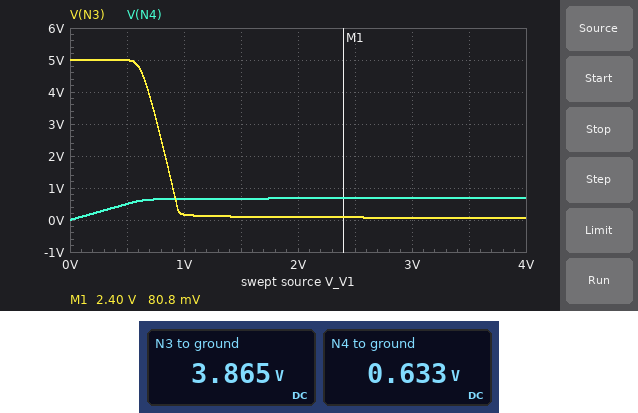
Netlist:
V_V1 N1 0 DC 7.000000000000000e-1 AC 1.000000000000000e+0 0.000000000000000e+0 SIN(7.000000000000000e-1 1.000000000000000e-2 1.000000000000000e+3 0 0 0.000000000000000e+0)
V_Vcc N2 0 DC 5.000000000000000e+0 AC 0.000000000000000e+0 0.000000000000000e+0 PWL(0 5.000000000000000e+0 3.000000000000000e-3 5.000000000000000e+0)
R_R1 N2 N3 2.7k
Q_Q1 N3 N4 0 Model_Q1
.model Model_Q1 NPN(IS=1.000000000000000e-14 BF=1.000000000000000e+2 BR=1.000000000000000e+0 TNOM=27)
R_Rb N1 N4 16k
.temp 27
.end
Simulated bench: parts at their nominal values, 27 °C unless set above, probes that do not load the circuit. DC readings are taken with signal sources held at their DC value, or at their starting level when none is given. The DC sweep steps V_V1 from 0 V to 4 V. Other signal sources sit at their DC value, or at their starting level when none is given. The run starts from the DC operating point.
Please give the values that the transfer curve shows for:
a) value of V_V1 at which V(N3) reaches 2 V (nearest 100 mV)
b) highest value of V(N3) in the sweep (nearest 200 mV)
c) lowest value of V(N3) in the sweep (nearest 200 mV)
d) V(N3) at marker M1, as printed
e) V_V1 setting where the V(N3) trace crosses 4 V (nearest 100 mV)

800 mV
5.0 V
0 V
80.8 mV
700 mV
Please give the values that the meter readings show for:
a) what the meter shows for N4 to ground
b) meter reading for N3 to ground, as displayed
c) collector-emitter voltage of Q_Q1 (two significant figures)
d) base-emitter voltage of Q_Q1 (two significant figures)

0.633 V
3.865 V
3.9 V
630 mV
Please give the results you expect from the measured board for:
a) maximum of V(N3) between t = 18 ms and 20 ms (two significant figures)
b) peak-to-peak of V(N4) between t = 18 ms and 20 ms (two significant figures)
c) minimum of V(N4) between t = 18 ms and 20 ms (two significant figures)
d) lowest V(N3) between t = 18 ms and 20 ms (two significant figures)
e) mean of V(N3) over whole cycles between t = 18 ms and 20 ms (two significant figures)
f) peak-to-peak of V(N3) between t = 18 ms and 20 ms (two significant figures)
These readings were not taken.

4.0 V
5.6 mV
630 mV
3.7 V
3.9 V
240 mV
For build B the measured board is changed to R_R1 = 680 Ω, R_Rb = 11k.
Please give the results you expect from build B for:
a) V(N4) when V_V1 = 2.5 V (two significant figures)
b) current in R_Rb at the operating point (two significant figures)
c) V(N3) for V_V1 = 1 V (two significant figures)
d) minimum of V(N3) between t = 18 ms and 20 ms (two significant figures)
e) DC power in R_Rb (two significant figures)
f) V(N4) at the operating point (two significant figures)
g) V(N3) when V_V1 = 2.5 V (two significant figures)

710 mV
5.5 µA
3.0 V
4.6 V
330 nW
640 mV
110 mV
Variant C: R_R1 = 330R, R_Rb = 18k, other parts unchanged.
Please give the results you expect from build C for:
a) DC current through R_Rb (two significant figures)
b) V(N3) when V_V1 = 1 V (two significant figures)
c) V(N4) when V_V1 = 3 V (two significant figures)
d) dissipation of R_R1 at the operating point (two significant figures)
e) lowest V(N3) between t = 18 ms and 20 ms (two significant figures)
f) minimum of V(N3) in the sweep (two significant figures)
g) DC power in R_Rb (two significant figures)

3.9 µA
4.4 V
720 mV
49 µW
4.9 V
160 mV
270 nW
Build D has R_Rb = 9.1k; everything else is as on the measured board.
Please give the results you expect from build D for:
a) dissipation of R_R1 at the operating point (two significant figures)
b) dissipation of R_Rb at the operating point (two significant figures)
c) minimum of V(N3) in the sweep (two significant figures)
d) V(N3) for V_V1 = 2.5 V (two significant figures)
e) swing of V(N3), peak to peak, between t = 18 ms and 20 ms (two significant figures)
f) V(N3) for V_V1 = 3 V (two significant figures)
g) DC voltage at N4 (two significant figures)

1.1 mW
360 nW
52 mV
65 mV
410 mV
59 mV
640 mV
